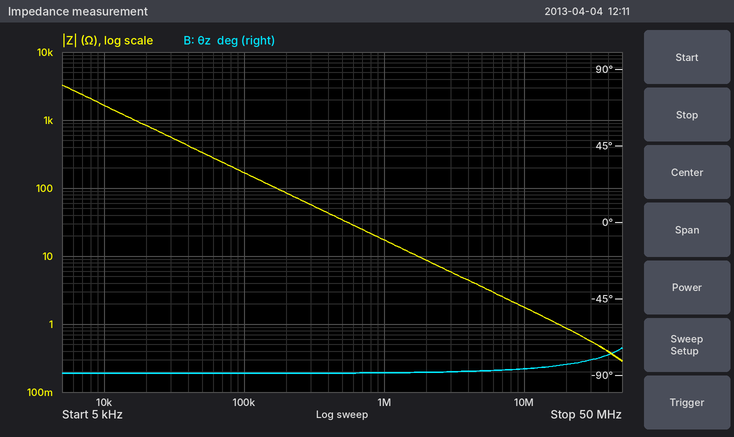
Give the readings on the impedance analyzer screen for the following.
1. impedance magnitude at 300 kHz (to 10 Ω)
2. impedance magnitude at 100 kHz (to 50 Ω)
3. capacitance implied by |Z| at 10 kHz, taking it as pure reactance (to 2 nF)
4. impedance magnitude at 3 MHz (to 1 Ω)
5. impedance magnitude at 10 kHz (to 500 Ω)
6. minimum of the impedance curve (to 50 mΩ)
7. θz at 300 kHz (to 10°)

60 Ω
150 Ω
10 nF
6 Ω
1.5 kΩ
300 mΩ
-90°
